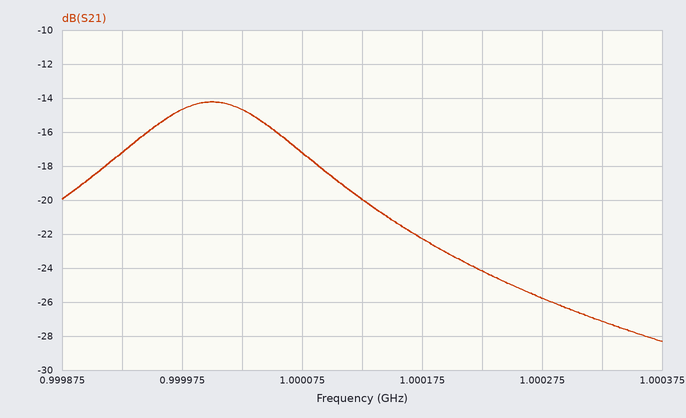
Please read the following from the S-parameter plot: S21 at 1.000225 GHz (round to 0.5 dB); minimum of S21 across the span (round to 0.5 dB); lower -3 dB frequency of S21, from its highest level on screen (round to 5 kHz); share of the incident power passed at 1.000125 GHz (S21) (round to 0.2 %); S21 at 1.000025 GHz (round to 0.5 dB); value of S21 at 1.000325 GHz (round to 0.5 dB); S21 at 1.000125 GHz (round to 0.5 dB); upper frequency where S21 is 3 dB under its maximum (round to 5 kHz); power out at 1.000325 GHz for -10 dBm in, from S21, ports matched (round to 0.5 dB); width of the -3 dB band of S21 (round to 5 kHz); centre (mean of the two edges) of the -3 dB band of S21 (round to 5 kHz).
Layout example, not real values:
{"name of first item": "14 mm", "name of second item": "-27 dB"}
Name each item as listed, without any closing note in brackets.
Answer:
{"S21 at 1.000225 GHz": "-24.0 dB", "minimum of S21 across the span": "-28.5 dB", "lower -3 dB frequency of S21, from its highest level on screen": "999.925 MHz", "share of the incident power passed at 1.000125 GHz (S21)": "1.0 %", "S21 at 1.000025 GHz": "-14.5 dB", "value of S21 at 1.000325 GHz": "-27.0 dB", "S21 at 1.000125 GHz": "-20.0 dB", "upper frequency where S21 is 3 dB under its maximum": "1.000075 GHz", "power out at 1.000325 GHz for -10 dBm in, from S21, ports matched": "-37.0 dBm", "width of the -3 dB band of S21": "150 kHz", "centre (mean of the two edges) of the -3 dB band of S21": "1.000000 GHz"}
